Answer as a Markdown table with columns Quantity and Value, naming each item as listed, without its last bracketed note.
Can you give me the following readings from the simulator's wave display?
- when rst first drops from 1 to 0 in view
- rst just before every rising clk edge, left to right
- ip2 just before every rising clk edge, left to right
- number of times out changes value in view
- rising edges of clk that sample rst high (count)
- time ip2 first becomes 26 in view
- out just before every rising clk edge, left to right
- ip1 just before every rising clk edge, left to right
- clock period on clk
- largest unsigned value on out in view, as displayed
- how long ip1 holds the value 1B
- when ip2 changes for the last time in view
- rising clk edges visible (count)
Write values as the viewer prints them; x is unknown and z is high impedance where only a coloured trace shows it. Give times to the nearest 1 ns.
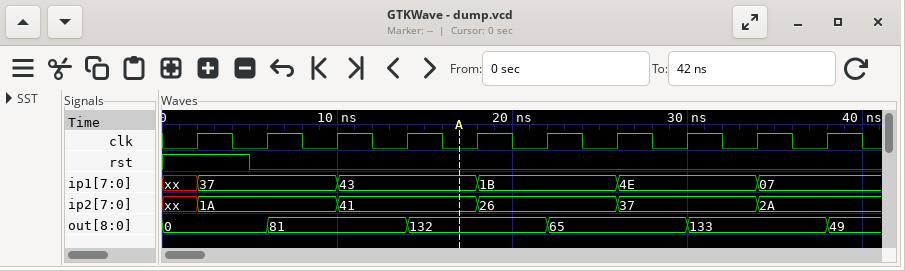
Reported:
| Quantity | Value |
|---|---|
| when rst first drops from 1 to 0 in view | 5 ns |
| rst just before every rising clk edge, left to right | 1 0 0 0 0 0 0 0 0 0 |
| ip2 just before every rising clk edge, left to right | xx, 1A, 1A, 41, 41, 26, 26, 37, 37, 2A |
| number of times out changes value in view | 5 |
| rising edges of clk that sample rst high | 1 |
| time ip2 first becomes 26 in view | 18 ns |
| out just before every rising clk edge, left to right | 0, 0, 81, 81, 132, 132, 65, 65, 133, 133 |
| ip1 just before every rising clk edge, left to right | xx, 37, 37, 43, 43, 1B, 1B, 4E, 4E, 07 |
| clock period on clk | 4 ns |
| largest unsigned value on out in view, as displayed | 133 |
| how long ip1 holds the value 1B | 8 ns |
| when ip2 changes for the last time in view | 34 ns |
| rising clk edges visible | 10 |
